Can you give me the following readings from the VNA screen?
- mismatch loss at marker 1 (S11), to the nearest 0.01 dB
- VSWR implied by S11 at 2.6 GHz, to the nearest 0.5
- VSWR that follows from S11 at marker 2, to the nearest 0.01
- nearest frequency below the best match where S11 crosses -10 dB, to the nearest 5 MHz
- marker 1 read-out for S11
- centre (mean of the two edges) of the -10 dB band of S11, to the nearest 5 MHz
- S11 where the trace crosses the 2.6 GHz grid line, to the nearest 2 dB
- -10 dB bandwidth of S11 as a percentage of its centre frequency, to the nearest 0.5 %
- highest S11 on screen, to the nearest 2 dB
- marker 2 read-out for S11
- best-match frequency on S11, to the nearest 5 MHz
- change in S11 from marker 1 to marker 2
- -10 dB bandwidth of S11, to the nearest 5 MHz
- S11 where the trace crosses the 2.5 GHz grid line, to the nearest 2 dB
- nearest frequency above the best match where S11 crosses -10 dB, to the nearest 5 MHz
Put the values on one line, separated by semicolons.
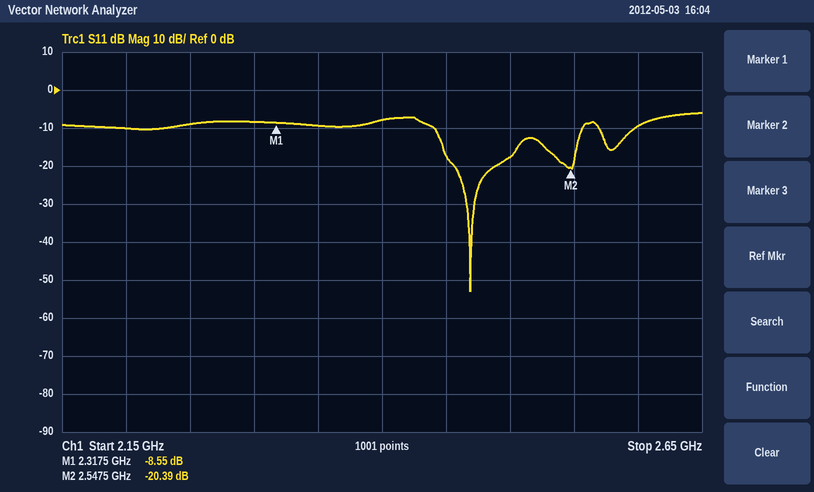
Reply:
0.65 dB; 2.0; 1.21; 2.440 GHz; -8.55 dB; 2.500 GHz; -10 dB; 4.5 %; -6 dB; -20.39 dB; 2.470 GHz; -11.84 dB; 115 MHz; -18 dB; 2.555 GHz
